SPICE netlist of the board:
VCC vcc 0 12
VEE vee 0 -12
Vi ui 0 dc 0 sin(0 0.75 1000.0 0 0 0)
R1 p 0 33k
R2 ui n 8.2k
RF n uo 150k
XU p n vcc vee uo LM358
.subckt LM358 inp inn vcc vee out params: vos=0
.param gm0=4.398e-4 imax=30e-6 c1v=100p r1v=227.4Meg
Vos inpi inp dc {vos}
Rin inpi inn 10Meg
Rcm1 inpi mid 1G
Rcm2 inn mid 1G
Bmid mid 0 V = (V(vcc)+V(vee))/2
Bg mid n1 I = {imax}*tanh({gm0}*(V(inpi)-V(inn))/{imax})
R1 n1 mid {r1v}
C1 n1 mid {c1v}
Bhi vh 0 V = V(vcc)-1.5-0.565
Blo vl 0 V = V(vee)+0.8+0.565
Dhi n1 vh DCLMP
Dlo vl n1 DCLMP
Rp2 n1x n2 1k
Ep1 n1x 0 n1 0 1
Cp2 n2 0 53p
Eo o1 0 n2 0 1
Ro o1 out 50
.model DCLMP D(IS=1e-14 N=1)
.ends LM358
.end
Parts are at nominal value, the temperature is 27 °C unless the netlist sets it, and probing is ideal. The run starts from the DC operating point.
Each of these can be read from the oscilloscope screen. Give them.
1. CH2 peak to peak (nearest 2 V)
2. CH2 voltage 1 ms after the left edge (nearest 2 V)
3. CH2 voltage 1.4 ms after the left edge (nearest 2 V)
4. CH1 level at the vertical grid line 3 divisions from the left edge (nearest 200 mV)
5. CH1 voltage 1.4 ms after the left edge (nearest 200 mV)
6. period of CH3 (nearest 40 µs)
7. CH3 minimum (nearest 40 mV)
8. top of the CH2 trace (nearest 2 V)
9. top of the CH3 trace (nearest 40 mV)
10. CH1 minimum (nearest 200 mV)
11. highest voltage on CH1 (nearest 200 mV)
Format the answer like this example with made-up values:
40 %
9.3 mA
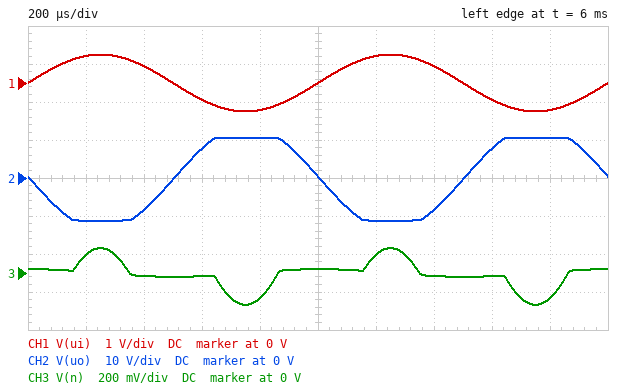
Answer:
22 V
0 V
-8 V
-400 mV
400 mV
1.00 ms
-160 mV
10 V
120 mV
-800 mV
800 mV
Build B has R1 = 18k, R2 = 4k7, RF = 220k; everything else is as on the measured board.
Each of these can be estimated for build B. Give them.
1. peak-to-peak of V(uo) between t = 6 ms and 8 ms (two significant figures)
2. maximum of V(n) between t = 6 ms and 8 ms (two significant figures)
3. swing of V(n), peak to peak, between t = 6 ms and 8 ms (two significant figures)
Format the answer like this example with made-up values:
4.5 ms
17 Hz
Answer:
22 V
500 mV
1.0 V
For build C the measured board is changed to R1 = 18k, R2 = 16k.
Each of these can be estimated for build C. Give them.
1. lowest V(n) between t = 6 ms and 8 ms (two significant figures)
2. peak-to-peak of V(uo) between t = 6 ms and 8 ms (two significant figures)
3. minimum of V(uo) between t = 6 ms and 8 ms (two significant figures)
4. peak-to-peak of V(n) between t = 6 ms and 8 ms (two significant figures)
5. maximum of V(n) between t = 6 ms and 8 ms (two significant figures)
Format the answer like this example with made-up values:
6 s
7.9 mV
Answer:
-10 mV
14 V
-7.0 V
20 mV
10 mV
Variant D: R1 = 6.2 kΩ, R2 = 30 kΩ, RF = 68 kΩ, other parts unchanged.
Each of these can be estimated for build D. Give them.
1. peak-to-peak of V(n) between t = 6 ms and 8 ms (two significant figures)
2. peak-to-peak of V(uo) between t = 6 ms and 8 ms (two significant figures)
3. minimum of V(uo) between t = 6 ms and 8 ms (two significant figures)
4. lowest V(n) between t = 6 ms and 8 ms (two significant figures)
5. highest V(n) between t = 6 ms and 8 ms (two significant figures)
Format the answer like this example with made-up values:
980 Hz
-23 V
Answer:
4.9 mV
3.4 V
-1.7 V
-2.4 mV
2.4 mV
